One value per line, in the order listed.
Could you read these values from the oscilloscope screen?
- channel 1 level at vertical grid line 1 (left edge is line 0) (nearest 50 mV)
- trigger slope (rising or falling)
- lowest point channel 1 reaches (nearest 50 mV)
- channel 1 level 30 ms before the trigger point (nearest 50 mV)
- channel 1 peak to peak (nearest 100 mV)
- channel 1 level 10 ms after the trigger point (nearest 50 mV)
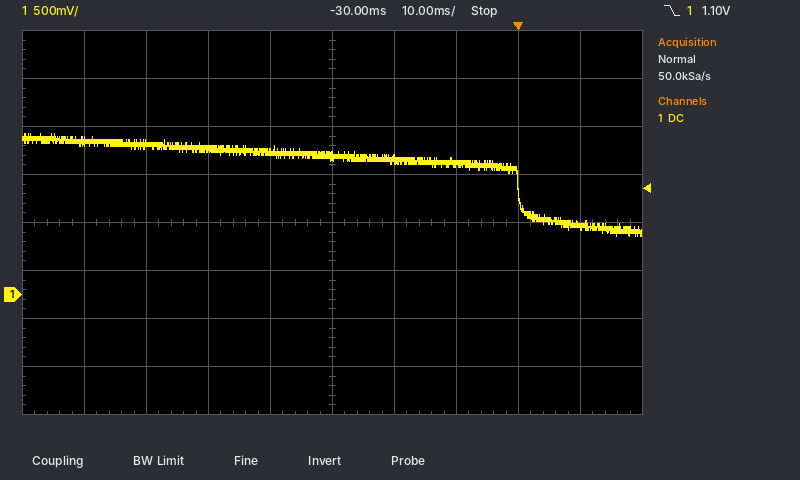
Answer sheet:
1.60 V
falling
600 mV
1.45 V
1.10 V
700 mV
